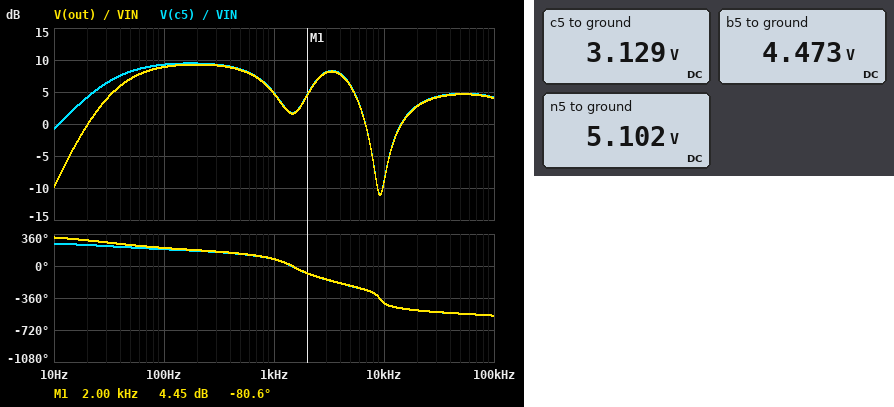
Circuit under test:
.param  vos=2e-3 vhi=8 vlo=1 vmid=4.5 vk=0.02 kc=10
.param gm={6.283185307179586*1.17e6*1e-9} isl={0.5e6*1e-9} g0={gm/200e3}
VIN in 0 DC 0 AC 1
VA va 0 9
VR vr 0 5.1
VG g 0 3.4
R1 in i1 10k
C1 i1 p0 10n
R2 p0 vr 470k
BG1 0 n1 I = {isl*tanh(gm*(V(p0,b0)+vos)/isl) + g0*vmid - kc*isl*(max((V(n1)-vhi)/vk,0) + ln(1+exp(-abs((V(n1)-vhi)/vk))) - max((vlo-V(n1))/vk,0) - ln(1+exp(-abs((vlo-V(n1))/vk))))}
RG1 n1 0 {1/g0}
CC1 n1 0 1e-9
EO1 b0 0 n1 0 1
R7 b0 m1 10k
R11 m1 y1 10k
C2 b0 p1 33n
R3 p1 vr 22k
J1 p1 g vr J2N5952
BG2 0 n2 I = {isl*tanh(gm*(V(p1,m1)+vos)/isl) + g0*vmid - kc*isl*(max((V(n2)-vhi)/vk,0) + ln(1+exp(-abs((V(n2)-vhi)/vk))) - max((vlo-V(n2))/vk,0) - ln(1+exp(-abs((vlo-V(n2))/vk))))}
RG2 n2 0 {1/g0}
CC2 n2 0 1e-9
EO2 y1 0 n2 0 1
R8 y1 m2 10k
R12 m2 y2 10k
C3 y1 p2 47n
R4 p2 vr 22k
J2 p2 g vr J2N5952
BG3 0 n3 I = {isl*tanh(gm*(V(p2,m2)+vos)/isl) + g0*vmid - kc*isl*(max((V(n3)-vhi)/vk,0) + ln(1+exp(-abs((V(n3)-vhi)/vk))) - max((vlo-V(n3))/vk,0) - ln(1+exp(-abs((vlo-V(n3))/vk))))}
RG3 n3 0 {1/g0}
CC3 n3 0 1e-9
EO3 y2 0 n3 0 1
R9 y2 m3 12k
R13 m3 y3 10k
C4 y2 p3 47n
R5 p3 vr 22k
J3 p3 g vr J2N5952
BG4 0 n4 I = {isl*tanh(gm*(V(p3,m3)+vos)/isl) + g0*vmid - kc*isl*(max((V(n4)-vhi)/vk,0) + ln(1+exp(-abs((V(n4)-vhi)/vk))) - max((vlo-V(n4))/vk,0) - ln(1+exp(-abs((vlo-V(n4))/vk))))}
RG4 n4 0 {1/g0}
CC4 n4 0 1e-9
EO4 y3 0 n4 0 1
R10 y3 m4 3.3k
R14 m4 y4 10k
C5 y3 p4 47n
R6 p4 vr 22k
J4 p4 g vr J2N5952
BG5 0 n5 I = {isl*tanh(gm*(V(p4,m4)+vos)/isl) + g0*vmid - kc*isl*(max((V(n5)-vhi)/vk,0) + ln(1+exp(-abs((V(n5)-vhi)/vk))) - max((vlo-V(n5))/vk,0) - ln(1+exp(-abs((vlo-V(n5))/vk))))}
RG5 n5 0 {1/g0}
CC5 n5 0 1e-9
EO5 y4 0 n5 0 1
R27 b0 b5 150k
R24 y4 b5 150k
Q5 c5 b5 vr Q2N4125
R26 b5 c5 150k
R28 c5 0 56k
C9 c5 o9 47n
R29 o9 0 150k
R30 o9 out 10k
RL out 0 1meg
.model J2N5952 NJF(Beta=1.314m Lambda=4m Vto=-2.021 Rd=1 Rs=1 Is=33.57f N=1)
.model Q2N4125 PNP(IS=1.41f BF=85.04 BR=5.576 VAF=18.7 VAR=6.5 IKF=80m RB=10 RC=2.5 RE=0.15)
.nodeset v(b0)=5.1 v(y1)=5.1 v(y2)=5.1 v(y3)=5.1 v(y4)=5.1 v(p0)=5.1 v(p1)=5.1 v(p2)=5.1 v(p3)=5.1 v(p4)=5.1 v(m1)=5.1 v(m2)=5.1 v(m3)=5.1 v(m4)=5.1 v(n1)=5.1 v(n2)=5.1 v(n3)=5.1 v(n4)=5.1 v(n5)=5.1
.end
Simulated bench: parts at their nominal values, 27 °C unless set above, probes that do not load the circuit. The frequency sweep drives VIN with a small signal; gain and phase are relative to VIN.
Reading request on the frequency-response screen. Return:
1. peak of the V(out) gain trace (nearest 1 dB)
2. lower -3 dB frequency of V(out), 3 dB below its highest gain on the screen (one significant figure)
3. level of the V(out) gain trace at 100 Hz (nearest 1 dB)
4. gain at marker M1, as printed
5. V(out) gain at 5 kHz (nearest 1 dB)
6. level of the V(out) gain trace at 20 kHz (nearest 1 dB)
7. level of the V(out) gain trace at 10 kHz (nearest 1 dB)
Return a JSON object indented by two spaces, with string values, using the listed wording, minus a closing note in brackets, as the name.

{
  "peak of the V(out) gain trace": "9 dB",
  "lower -3 dB frequency of V(out), 3 dB below its highest gain on the screen": "40 Hz",
  "level of the V(out) gain trace at 100 Hz": "9 dB",
  "gain at marker M1, as printed": "4.45 dB",
  "V(out) gain at 5 kHz": "6 dB",
  "level of the V(out) gain trace at 20 kHz": "3 dB",
  "level of the V(out) gain trace at 10 kHz": "-9 dB"
}
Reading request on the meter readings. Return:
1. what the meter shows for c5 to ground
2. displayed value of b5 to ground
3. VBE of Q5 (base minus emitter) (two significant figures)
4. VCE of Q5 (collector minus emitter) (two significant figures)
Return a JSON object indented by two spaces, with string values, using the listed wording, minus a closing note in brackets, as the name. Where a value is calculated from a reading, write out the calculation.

{
  "what the meter shows for c5 to ground": "3.129 V",
  "displayed value of b5 to ground": "4.473 V",
  "VBE of Q5 (base minus emitter)": "4.473 V - 5.1 V = -630 mV",
  "VCE of Q5 (collector minus emitter)": "3.129 V - 5.1 V = -2.0 V"
}
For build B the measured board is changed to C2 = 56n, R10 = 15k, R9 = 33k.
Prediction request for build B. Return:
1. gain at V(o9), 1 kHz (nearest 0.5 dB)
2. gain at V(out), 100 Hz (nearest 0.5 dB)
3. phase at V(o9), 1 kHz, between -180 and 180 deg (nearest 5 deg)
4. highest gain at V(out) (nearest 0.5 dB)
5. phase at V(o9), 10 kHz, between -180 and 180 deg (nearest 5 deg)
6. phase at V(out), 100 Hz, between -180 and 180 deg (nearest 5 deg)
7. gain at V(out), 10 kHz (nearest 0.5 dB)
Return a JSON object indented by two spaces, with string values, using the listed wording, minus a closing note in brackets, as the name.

{
  "gain at V(o9), 1 kHz": "-4.0 dB",
  "gain at V(out), 100 Hz": "-0.5 dB",
  "phase at V(o9), 1 kHz, between -180 and 180 deg": "-170 deg",
  "highest gain at V(out)": "4.5 dB",
  "phase at V(o9), 10 kHz, between -180 and 180 deg": "-130 deg",
  "phase at V(out), 100 Hz, between -180 and 180 deg": "-150 deg",
  "gain at V(out), 10 kHz": "0 dB"
}
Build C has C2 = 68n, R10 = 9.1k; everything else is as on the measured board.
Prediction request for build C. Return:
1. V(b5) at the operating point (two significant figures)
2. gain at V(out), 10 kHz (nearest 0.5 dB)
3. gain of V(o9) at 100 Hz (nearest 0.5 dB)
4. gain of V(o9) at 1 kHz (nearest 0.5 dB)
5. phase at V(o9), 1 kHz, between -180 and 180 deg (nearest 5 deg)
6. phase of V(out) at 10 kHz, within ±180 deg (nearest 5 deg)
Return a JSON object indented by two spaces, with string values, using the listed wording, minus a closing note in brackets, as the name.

{
  "V(b5) at the operating point": "4.5 V",
  "gain at V(out), 10 kHz": "-1.0 dB",
  "gain of V(o9) at 100 Hz": "3.5 dB",
  "gain of V(o9) at 1 kHz": "-12.5 dB",
  "phase at V(o9), 1 kHz, between -180 and 180 deg": "115 deg",
  "phase of V(out) at 10 kHz, within ±180 deg": "-120 deg"
}
